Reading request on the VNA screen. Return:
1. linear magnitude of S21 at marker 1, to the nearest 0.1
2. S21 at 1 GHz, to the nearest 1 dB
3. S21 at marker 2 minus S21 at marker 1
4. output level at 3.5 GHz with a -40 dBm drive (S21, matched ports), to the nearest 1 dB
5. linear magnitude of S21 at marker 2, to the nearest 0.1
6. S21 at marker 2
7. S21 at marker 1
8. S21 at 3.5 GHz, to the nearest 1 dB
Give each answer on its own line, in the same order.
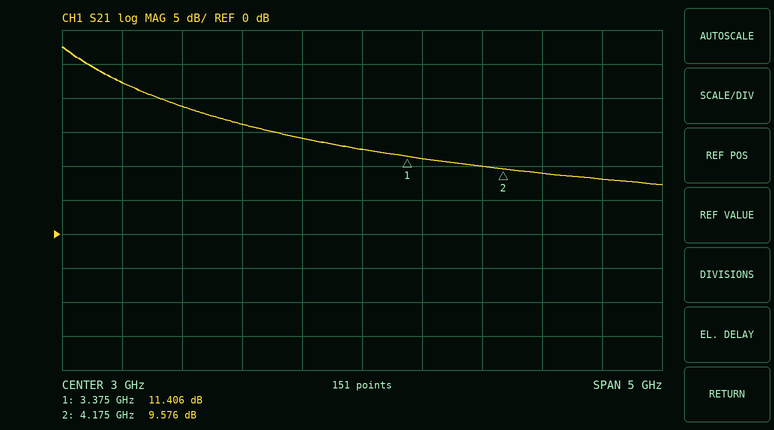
3.7
22 dB
-1.830 dB
-29 dBm
3.0
9.576 dB
11.406 dB
11 dB
